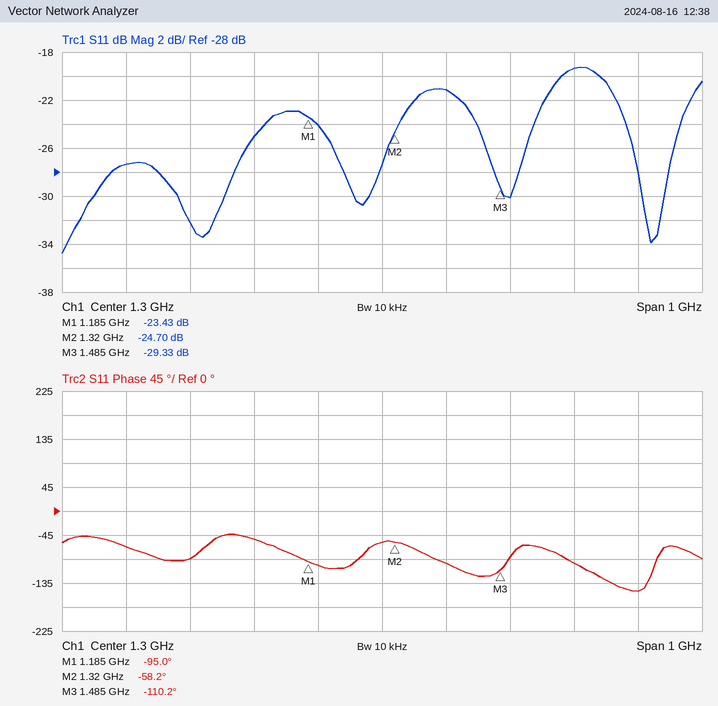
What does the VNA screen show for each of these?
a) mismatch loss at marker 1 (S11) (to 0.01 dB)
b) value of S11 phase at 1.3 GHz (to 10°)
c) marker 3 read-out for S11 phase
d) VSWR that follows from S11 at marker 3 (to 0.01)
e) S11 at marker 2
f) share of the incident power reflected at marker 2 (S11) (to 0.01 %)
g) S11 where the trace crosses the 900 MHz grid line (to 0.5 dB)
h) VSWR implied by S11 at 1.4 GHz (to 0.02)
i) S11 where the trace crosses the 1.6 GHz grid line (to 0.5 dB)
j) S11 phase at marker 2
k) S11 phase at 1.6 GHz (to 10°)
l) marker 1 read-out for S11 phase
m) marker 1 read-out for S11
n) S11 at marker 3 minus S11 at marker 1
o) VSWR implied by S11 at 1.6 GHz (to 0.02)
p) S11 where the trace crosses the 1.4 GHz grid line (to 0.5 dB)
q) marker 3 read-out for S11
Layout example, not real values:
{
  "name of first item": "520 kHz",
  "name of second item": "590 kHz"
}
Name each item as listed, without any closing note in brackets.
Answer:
{
  "mismatch loss at marker 1 (S11)": "0.02 dB",
  "value of S11 phase at 1.3 GHz": "-60°",
  "marker 3 read-out for S11 phase": "-110.2°",
  "VSWR that follows from S11 at marker 3": "1.07",
  "S11 at marker 2": "-24.70 dB",
  "share of the incident power reflected at marker 2 (S11)": "0.34 %",
  "S11 where the trace crosses the 900 MHz grid line": "-27.5 dB",
  "VSWR implied by S11 at 1.4 GHz": "1.20",
  "S11 where the trace crosses the 1.6 GHz grid line": "-19.5 dB",
  "S11 phase at marker 2": "-58.2°",
  "S11 phase at 1.6 GHz": "-100°",
  "marker 1 read-out for S11 phase": "-95.0°",
  "marker 1 read-out for S11": "-23.43 dB",
  "S11 at marker 3 minus S11 at marker 1": "-5.90 dB",
  "VSWR implied by S11 at 1.6 GHz": "1.24",
  "S11 where the trace crosses the 1.4 GHz grid line": "-21.0 dB",
  "marker 3 read-out for S11": "-29.33 dB"
}
